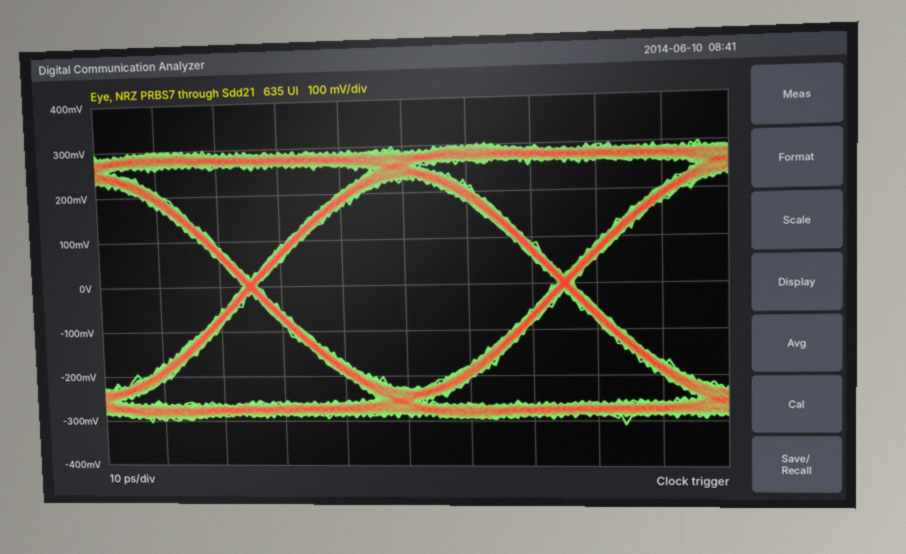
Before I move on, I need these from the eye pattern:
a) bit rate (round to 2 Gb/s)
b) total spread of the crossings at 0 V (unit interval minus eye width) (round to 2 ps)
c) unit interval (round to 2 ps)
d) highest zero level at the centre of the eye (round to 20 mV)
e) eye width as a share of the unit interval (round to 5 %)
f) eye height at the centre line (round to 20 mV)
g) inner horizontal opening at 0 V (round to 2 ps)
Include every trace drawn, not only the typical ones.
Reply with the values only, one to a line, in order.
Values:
20 Gb/s
2 ps
50 ps
-220 mV
95 %
460 mV
48 ps
